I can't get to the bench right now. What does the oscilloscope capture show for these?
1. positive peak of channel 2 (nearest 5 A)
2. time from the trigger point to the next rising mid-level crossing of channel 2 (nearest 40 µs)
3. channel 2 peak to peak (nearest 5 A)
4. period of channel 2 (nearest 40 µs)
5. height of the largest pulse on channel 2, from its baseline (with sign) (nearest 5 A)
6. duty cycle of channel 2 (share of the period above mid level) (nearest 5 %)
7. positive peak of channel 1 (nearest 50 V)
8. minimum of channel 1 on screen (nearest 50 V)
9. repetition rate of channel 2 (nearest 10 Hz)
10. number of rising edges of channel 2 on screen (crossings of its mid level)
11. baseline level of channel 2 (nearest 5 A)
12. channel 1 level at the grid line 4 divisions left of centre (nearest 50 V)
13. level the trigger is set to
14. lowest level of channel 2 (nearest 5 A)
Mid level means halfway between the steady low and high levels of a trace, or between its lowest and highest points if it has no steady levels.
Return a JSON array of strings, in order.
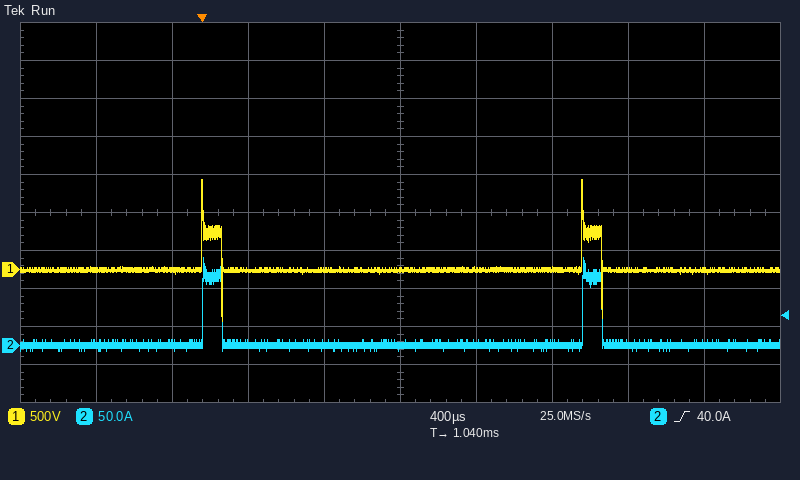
["115 A", "2.00 ms", "125 A", "2.00 ms", "+115 A", "5 %", "1.20 kV", "-700 V", "500 Hz", "2", "0 A", "0 V", "40.0 A", "-10 A"]
